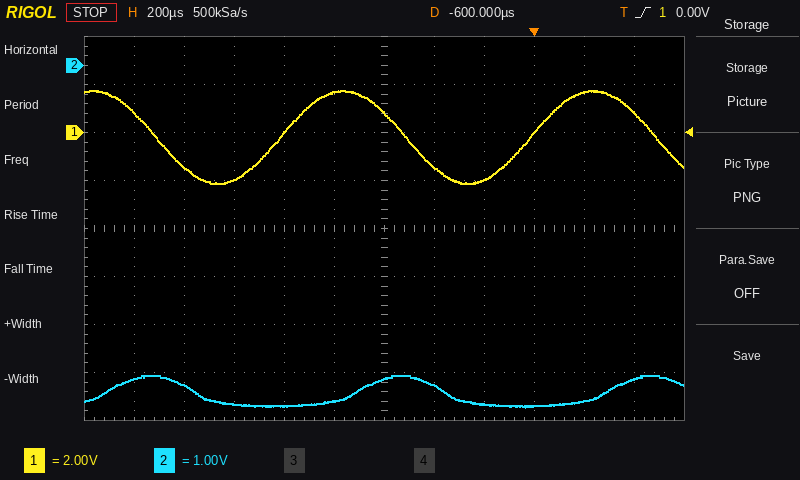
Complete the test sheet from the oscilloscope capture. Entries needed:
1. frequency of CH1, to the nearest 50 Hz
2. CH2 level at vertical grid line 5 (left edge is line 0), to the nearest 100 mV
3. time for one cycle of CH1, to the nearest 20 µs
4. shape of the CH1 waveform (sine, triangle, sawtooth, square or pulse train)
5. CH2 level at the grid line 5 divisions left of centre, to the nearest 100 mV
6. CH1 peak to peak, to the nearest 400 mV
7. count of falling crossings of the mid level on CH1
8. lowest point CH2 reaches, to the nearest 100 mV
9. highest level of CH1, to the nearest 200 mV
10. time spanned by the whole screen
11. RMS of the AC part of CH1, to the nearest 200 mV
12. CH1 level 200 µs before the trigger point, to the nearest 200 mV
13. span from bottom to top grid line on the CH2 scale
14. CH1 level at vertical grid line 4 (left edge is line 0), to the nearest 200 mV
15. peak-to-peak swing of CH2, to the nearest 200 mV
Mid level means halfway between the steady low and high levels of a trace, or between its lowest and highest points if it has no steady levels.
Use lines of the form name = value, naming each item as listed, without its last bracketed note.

frequency of CH1, to the nearest 50 Hz = 1.00 kHz
CH2 level at vertical grid line 5 (left edge is line 0), to the nearest 100 mV = -7.0 V
time for one cycle of CH1, to the nearest 20 µs = 1.00 ms
shape of the CH1 waveform = sine
CH2 level at the grid line 5 divisions left of centre, to the nearest 100 mV = -6.5 V
CH1 peak to peak, to the nearest 400 mV = 4.0 V
count of falling crossings of the mid level on CH1 = 3
lowest point CH2 reaches, to the nearest 100 mV = -7.1 V
highest level of CH1, to the nearest 200 mV = 1.8 V
time spanned by the whole screen = 2.4 ms
RMS of the AC part of CH1, to the nearest 200 mV = 1.4 V
CH1 level 200 µs before the trigger point, to the nearest 200 mV = -2.0 V
span from bottom to top grid line on the CH2 scale = 8 V
CH1 level at vertical grid line 4 (left edge is line 0), to the nearest 200 mV = 0.0 V
peak-to-peak swing of CH2, to the nearest 200 mV = 600 mV
